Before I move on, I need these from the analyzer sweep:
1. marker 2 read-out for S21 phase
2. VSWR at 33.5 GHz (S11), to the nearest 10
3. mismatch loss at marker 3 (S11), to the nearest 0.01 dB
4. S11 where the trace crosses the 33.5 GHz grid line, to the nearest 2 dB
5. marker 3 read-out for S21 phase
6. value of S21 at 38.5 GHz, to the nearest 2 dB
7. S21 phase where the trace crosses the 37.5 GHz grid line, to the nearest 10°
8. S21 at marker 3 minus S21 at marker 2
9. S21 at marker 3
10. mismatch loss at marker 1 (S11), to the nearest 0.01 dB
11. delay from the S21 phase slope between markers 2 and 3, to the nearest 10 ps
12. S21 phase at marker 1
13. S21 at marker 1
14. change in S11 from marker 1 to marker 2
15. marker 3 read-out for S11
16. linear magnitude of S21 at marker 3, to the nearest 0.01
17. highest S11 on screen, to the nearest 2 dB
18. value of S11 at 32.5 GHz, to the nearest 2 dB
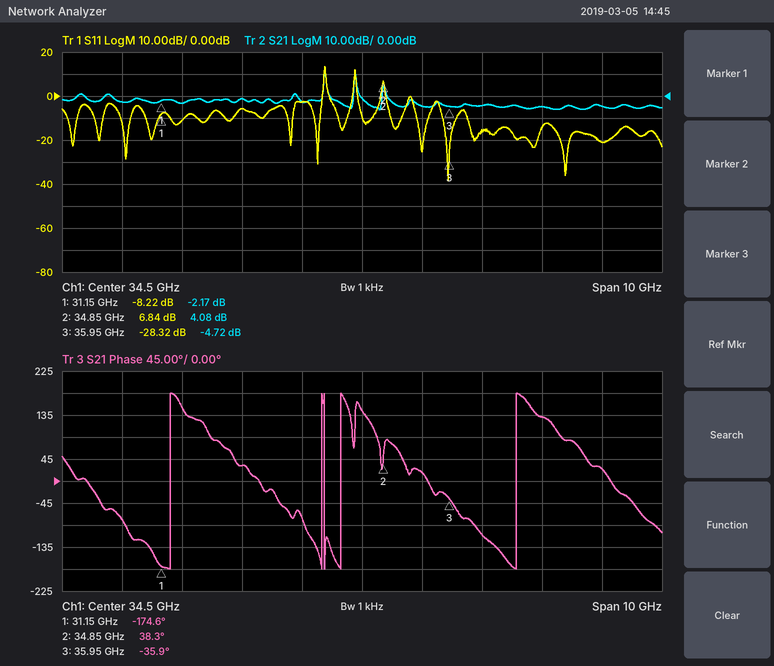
38.3°
10
0.01 dB
-2 dB
-35.9°
-4 dB
130°
-8.80 dB
-4.72 dB
0.71 dB
190 ps
-174.6°
-2.17 dB
15.06 dB
-28.32 dB
0.58
14 dB
-6 dB
